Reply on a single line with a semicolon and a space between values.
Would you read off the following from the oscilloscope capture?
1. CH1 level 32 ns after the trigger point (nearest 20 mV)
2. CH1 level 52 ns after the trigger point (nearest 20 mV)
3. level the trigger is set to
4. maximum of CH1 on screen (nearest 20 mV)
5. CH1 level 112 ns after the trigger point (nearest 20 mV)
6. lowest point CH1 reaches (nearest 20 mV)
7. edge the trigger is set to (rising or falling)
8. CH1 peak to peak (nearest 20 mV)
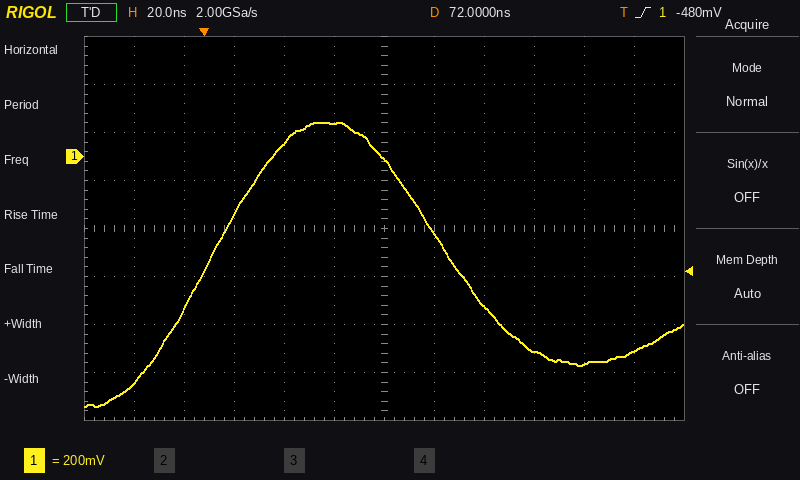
60 mV; 140 mV; -480 mV; 140 mV; -620 mV; -1.04 V; rising; 1.18 V
